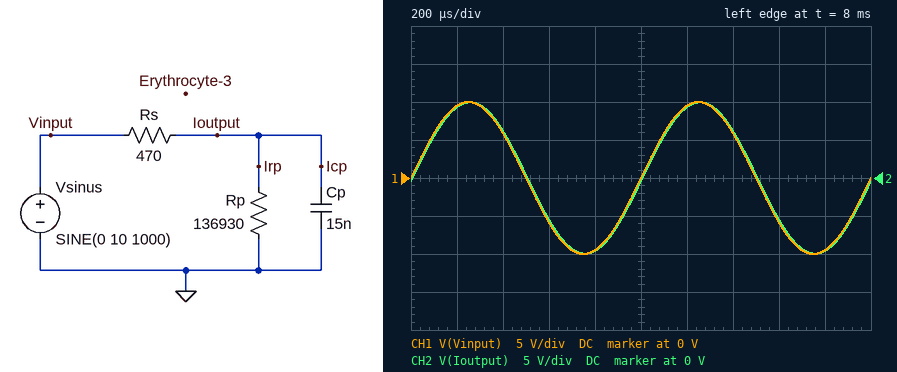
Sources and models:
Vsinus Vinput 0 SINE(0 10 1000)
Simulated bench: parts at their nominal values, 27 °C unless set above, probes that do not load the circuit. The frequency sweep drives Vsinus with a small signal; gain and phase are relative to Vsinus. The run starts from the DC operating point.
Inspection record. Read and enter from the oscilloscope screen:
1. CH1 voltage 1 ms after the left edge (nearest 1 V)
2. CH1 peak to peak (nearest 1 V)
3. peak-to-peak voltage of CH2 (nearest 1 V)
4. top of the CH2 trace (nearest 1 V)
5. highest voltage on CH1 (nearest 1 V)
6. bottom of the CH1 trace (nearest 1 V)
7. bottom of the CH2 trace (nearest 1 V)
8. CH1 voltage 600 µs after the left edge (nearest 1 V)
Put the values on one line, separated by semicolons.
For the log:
0 V; 20 V; 20 V; 10 V; 10 V; -10 V; -10 V; -6 V
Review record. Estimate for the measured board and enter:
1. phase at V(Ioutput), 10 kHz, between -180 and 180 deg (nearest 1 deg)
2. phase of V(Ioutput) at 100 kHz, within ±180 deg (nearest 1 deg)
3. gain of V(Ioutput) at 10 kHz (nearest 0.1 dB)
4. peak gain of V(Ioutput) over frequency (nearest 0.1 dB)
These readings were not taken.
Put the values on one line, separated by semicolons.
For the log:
-24 deg; -77 deg; -0.8 dB; 0 dB
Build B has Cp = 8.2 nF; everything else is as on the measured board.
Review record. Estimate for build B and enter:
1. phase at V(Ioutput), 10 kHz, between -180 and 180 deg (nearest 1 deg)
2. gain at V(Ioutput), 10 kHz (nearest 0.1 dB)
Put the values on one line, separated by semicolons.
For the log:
-14 deg; -0.3 dB
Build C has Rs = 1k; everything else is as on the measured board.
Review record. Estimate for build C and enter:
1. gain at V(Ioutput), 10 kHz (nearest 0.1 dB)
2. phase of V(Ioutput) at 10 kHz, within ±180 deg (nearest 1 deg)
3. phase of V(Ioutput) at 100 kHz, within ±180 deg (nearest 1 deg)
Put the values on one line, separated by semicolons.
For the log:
-2.8 dB; -43 deg; -84 deg
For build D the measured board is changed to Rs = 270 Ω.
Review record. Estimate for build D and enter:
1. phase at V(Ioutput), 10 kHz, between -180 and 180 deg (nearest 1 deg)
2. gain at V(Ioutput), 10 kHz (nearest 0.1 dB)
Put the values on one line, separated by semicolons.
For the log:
-14 deg; -0.3 dB
